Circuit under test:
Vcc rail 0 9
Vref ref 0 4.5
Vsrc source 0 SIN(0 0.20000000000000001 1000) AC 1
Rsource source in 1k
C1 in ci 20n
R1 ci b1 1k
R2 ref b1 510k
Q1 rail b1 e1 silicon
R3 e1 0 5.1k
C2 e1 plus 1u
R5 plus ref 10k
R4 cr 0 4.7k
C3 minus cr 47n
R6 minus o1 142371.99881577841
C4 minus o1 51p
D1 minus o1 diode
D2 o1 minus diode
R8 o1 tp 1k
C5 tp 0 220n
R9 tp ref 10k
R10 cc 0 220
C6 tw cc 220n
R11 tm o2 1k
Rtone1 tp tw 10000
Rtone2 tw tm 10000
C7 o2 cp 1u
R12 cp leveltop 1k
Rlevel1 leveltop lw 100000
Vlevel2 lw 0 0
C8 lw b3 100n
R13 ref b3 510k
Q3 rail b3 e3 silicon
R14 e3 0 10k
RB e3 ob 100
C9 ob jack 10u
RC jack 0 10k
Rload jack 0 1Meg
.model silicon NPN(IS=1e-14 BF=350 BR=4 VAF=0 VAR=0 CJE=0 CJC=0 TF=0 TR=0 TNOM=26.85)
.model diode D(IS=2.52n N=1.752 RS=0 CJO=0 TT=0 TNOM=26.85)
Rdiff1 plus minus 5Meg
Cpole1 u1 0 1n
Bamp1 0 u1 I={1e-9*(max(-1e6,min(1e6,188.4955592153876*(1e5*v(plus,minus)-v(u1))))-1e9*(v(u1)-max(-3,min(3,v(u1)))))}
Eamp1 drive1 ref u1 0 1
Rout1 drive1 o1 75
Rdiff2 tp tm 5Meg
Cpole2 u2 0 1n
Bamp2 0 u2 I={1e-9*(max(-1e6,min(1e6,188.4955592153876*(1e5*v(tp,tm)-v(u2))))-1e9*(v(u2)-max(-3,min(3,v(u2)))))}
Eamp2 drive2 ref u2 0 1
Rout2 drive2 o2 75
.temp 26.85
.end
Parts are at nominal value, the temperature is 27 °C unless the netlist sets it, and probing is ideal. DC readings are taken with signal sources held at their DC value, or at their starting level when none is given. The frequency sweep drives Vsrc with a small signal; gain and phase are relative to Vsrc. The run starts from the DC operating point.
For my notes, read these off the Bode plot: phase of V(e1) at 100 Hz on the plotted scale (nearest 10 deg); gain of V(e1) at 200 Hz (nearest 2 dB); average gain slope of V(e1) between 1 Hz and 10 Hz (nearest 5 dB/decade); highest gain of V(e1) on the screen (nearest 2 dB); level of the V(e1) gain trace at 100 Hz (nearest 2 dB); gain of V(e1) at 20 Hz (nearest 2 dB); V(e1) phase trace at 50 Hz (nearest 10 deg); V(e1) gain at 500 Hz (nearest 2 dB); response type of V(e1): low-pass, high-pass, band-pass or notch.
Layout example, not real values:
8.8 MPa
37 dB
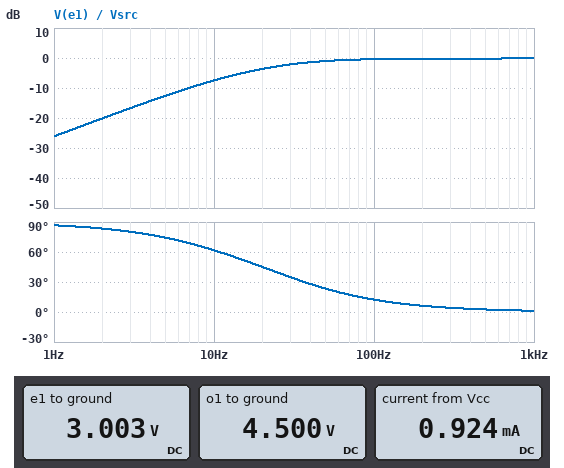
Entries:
10 deg
0 dB
20 dB/decade
0 dB
0 dB
-4 dB
20 deg
0 dB
high-pass
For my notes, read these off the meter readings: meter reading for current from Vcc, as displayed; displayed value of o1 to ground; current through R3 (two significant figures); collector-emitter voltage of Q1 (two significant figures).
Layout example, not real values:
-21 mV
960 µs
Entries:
0.924 mA
4.500 V
590 µA
6.0 V
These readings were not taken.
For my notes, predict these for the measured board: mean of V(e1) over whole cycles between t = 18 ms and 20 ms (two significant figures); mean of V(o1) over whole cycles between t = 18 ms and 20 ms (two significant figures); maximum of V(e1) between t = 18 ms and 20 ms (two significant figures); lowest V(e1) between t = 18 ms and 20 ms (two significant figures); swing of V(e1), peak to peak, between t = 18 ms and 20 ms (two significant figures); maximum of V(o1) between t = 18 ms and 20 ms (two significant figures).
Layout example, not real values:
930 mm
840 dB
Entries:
3.0 V
4.5 V
3.2 V
2.8 V
390 mV
5.1 V
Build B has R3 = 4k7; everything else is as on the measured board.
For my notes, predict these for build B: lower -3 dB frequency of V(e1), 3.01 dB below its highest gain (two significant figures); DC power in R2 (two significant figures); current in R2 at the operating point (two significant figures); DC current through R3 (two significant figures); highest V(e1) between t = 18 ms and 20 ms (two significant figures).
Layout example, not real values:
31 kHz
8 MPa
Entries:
23 Hz
1.6 µW
1.8 µA
630 µA
3.1 V
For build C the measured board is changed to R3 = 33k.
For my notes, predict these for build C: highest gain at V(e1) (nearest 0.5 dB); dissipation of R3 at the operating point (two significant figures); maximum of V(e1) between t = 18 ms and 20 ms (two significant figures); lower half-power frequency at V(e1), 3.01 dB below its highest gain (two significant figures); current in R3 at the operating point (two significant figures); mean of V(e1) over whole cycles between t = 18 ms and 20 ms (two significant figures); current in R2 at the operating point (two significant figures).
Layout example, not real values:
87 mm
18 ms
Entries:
-0.5 dB
420 µW
3.9 V
18 Hz
110 µA
3.7 V
320 nA
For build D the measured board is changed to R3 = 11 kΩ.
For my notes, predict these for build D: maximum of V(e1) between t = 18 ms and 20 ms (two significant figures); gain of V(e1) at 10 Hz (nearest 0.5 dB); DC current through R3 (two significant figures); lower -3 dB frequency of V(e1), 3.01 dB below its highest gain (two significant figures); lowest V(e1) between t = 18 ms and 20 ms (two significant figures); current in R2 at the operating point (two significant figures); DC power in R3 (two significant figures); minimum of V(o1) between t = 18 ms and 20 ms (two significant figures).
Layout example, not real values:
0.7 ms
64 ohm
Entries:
3.6 V
-6.5 dB
310 µA
20 Hz
3.2 V
890 nA
1.1 mW
3.9 V
